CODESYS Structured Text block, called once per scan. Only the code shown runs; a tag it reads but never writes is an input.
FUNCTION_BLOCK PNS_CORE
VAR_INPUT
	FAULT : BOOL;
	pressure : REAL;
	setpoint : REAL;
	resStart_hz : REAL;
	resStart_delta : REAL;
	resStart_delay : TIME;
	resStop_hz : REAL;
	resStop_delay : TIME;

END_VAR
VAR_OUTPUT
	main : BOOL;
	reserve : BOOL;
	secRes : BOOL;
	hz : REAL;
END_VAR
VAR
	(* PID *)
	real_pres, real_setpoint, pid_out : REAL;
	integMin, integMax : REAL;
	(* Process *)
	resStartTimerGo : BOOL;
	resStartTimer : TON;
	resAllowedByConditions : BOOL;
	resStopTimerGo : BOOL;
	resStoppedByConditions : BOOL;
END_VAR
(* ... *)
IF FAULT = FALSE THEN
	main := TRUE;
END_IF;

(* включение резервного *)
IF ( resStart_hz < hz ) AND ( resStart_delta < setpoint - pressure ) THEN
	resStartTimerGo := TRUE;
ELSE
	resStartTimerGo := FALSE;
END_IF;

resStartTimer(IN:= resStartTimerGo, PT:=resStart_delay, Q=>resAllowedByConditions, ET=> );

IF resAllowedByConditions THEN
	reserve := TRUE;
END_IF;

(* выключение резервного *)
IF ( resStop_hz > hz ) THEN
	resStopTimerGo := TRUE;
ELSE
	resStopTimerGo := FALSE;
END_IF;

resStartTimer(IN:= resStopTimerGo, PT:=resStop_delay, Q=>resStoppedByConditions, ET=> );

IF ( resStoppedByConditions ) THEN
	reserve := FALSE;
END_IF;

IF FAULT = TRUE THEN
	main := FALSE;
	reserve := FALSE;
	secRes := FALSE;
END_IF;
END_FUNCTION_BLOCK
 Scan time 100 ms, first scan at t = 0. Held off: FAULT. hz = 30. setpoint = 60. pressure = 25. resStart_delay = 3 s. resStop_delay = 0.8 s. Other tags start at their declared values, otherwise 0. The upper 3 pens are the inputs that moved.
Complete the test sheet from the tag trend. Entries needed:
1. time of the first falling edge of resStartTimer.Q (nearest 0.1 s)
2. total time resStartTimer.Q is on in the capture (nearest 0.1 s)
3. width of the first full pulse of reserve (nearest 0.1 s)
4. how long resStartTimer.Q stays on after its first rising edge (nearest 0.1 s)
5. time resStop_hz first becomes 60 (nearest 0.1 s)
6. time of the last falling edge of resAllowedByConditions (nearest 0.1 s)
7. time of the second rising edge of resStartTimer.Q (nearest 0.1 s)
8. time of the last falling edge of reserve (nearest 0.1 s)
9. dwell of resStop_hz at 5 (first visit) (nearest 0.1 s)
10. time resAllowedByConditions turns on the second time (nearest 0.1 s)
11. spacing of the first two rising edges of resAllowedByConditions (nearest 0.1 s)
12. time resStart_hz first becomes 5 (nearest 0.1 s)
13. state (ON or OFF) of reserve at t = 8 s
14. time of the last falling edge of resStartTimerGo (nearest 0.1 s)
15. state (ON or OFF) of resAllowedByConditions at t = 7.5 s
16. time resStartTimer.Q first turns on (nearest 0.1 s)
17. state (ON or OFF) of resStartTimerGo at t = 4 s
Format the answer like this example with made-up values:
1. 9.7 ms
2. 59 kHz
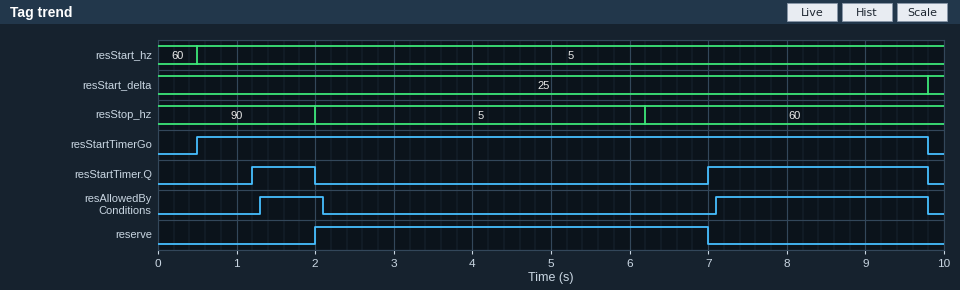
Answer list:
1. 2.0 s
2. 3.6 s
3. 5.0 s
4. 0.8 s
5. 6.2 s
6. 9.8 s
7. 7.0 s
8. 7.0 s
9. 4.2 s
10. 7.1 s
11. 5.8 s
12. 0.5 s
13. OFF
14. 9.8 s
15. ON
16. 1.2 s
17. ON
